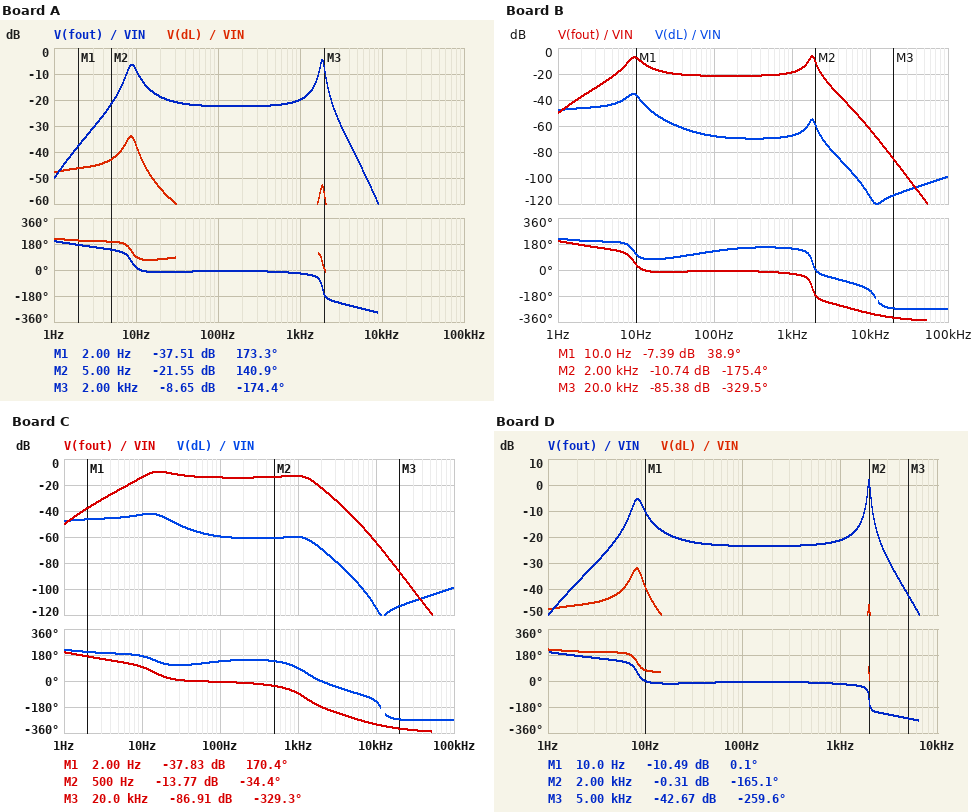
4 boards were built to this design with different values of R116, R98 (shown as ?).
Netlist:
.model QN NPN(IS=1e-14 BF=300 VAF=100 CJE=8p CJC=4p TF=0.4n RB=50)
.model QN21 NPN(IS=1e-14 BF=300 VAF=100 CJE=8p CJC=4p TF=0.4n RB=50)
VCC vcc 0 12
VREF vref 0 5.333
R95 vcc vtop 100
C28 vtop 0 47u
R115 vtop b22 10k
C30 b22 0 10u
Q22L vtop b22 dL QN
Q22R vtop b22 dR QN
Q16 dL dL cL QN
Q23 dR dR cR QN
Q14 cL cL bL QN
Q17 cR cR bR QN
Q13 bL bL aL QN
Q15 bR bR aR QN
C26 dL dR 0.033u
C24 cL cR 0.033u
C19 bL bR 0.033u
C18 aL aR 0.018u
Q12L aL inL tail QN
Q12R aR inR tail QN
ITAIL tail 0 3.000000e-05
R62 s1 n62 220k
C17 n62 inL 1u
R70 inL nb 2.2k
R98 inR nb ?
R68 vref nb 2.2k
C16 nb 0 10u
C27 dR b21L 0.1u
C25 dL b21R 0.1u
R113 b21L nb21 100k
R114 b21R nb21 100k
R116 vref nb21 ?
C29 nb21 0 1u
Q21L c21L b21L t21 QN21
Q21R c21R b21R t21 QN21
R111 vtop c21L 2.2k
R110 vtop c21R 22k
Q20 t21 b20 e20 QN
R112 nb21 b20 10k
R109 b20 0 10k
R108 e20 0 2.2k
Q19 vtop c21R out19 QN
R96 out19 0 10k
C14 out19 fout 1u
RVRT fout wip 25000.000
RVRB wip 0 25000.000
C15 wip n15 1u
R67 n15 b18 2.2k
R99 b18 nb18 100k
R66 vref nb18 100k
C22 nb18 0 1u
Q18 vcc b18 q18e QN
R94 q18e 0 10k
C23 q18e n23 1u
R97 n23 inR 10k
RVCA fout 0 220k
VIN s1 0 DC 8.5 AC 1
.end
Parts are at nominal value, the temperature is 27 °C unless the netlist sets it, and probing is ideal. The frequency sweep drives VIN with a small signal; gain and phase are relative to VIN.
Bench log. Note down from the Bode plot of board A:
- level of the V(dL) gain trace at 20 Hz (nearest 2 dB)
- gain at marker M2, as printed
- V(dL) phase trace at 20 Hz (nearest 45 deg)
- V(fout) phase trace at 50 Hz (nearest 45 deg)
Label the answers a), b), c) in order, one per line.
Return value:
a) -54 dB
b) -21.55 dB
c) 90 deg
d) 0 deg
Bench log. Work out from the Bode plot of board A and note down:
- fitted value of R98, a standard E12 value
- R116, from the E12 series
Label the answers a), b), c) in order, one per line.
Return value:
a) 3.9 kΩ
b) 5.6 kΩ
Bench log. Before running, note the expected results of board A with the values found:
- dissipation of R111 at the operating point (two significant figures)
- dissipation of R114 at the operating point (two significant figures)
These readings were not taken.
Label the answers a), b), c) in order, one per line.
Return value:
a) 240 µW
b) 110 nW
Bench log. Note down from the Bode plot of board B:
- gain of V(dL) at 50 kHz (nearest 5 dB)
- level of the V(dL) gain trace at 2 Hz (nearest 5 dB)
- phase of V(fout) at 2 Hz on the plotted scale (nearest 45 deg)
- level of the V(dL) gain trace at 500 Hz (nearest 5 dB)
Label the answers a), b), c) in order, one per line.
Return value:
a) -105 dB
b) -45 dB
c) 180 deg
d) -70 dB
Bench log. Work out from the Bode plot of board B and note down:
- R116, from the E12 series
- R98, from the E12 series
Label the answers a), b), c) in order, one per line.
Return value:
a) 4.7 kΩ
b) 3.3 kΩ
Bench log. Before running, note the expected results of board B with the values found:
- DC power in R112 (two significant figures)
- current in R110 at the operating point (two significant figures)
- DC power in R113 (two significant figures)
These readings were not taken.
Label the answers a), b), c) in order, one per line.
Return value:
a) 470 µW
b) 330 µA
c) 120 nW
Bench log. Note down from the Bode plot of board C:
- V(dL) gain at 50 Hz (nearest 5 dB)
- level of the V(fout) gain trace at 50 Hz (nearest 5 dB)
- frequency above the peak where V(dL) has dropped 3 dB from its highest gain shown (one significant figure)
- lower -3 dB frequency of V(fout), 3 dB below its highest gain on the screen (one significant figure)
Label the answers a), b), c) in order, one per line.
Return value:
a) -55 dB
b) -15 dB
c) 20 Hz
d) 10 Hz
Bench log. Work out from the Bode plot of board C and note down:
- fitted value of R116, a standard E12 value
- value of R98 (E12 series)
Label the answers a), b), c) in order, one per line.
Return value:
a) 8.2 kΩ
b) 1 kΩ
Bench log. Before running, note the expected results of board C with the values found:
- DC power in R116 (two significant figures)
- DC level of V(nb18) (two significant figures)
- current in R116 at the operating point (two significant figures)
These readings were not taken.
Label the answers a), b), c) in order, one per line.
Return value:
a) 300 µW
b) 5.2 V
c) 190 µA
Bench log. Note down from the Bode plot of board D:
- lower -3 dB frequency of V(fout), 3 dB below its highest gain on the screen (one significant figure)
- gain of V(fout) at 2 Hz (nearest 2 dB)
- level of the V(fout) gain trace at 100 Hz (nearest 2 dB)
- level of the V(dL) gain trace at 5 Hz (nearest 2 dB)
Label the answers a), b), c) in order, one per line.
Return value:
a) 2 kHz
b) -38 dB
c) -24 dB
d) -42 dB
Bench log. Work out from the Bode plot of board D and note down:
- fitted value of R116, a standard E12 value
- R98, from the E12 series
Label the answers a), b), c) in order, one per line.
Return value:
a) 5.6 kΩ
b) 4.7 kΩ
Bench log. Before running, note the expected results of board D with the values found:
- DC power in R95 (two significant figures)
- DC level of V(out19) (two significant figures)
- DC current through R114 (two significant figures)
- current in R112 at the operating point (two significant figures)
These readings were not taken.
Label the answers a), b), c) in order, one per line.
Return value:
a) 120 µW
b) 4.4 V
c) 1.0 µA
d) 210 µA
